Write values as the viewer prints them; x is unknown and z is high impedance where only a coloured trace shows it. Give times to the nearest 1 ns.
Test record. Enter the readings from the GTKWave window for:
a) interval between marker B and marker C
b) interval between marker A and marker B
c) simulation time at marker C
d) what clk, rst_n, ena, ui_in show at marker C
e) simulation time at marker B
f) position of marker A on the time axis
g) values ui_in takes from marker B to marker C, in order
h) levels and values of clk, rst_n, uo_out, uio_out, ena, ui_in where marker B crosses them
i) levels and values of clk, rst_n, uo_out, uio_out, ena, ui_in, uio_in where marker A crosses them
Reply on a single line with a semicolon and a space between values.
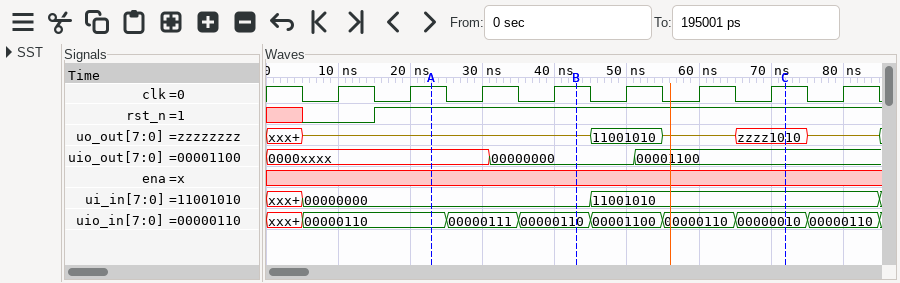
29 ns; 20 ns; 72 ns; clk=1, rst_n=1, ena=x, ui_in=11001010; 43 ns; 23 ns; 00000000, 11001010; clk=1, rst_n=1, uo_out=z, uio_out=00000000, ena=x, ui_in=00000000; clk=1, rst_n=1, uo_out=z, uio_out=0000xxxx, ena=x, ui_in=00000000, uio_in=00000110
